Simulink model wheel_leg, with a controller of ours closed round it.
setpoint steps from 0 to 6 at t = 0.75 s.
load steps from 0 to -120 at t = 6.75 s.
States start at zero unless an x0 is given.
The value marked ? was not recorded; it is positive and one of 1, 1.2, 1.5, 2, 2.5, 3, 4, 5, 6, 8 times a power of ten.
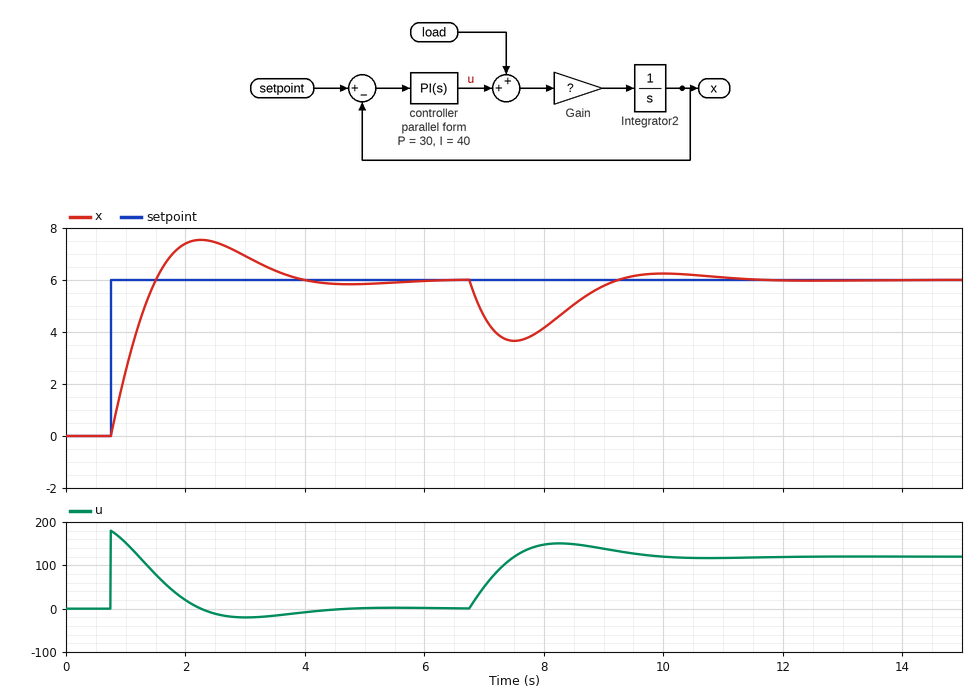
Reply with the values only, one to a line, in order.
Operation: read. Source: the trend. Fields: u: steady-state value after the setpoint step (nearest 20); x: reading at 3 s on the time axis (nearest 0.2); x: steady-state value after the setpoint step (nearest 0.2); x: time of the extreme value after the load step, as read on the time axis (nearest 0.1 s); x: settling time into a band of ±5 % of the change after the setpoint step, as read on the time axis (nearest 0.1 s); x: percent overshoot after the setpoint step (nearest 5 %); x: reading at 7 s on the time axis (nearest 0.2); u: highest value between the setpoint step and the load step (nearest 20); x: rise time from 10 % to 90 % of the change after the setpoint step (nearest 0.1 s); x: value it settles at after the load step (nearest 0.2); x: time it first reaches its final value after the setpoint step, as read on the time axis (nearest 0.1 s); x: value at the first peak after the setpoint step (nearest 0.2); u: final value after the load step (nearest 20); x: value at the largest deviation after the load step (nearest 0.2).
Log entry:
0
7.0
6.0
7.5 s
3.6 s
25 %
4.6
180
0.6 s
6.0
1.5 s
7.6
120
3.6
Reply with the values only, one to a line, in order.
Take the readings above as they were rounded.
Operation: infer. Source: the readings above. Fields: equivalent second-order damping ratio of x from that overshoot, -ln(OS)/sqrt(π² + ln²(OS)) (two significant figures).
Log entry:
0.40
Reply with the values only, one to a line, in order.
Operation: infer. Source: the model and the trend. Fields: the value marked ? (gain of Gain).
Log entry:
0.06
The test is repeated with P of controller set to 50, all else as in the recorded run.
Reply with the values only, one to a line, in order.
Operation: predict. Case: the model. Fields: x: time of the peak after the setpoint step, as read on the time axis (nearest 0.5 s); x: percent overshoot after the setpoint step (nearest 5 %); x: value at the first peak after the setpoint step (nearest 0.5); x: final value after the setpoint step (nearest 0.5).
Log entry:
2.0 s
15 %
7.0
6.0
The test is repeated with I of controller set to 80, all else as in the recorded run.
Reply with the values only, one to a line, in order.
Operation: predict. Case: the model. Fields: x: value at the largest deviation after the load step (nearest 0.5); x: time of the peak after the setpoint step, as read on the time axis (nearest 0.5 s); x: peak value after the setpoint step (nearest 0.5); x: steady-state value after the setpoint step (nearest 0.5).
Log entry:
4.0
2.0 s
8.0
6.0
